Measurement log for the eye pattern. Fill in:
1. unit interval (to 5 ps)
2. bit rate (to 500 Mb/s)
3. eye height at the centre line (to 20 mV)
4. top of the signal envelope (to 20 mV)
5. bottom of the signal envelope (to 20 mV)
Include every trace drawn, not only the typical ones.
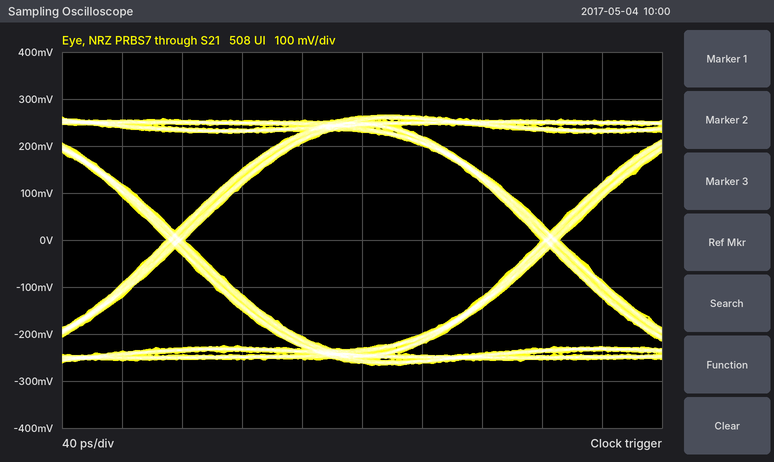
250 ps
4.0 Gb/s
460 mV
260 mV
-260 mV
